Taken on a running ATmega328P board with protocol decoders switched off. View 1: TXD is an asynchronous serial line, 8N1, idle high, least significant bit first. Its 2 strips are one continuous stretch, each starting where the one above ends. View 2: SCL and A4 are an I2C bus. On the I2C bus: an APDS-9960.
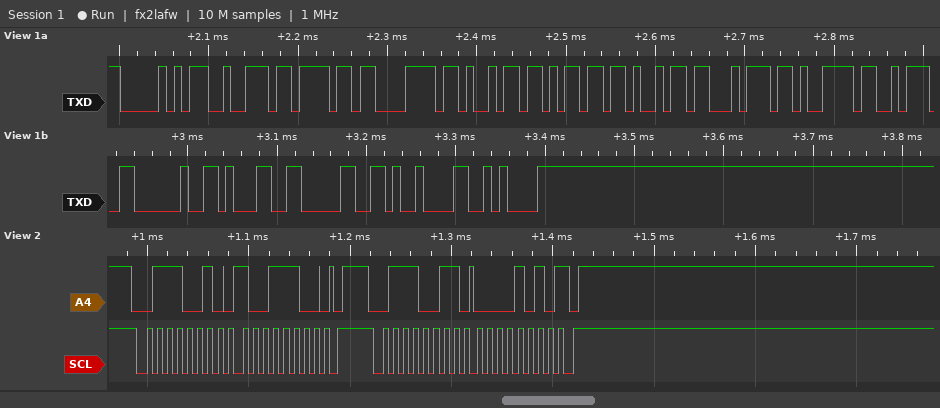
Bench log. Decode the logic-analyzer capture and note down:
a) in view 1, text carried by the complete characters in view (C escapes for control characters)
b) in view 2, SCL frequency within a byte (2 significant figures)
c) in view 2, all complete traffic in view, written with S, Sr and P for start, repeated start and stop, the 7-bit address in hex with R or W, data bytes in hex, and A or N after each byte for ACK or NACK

"Proximity: 10\t\n"
100 kHz
S 39W A 9C A P S 39R A 0A N P
